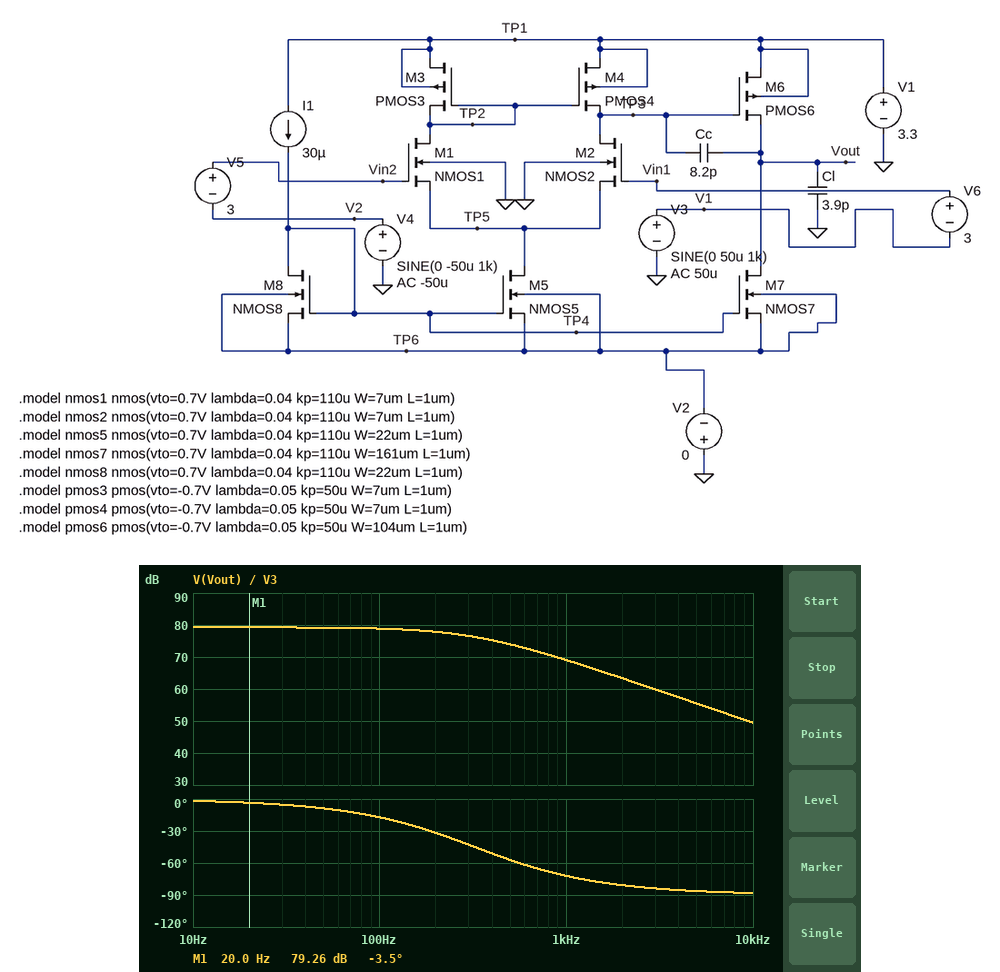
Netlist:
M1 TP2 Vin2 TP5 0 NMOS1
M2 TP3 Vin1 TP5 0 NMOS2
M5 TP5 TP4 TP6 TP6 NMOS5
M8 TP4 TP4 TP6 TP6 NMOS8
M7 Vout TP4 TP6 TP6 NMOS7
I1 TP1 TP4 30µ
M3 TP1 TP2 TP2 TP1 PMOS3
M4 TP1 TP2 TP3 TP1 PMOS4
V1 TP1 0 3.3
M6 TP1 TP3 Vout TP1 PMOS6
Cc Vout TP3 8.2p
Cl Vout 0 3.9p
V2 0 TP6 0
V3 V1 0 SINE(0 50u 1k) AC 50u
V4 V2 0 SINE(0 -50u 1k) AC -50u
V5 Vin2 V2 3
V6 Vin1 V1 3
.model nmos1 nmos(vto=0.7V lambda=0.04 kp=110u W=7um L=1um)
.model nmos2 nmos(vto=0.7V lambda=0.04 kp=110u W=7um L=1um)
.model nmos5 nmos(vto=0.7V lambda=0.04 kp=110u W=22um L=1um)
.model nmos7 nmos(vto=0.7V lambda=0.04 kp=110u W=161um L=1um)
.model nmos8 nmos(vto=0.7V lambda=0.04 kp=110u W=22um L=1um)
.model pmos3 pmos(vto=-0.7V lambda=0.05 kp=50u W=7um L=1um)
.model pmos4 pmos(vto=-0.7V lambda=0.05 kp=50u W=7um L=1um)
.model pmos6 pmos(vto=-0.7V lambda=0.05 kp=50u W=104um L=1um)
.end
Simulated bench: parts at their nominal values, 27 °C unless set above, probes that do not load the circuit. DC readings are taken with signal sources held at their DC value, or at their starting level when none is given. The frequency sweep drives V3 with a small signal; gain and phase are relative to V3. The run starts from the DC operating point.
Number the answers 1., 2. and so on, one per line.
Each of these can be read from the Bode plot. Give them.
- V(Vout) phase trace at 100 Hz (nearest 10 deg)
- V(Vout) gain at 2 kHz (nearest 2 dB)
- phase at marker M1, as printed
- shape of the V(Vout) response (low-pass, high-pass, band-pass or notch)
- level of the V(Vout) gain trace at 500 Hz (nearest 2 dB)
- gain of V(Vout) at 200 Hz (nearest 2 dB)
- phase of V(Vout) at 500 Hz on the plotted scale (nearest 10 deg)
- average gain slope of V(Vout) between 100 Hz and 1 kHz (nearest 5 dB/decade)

1. -20 deg
2. 64 dB
3. -3.5 deg
4. low-pass
5. 74 dB
6. 78 dB
7. -60 deg
8. -10 dB/decade
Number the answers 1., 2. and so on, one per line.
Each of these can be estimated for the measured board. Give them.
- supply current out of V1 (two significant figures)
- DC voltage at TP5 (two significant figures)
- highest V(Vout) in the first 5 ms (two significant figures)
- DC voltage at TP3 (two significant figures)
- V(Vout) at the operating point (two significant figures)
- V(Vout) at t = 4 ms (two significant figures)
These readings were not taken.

1. 290 µA
2. 2.1 V
3. 2.8 V
4. 2.3 V
5. 2.4 V
6. 2.1 V
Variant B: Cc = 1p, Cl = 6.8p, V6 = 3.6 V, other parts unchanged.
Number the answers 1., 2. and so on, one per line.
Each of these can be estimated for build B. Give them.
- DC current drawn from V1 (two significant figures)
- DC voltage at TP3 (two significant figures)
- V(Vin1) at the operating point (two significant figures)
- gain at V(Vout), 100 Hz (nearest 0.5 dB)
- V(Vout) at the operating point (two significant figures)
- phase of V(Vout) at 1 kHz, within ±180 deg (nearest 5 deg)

1. 300 µA
2. 2.1 V
3. 3.6 V
4. -40.0 dB
5. 3.2 V
6. 0 deg
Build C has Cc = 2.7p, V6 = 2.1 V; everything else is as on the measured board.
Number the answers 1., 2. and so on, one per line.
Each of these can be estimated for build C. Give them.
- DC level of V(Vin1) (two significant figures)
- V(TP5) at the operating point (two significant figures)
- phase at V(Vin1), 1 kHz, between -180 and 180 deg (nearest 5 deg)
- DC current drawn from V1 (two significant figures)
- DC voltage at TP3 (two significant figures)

1. 2.1 V
2. 2.0 V
3. 0 deg
4. 61 µA
5. 3.3 V
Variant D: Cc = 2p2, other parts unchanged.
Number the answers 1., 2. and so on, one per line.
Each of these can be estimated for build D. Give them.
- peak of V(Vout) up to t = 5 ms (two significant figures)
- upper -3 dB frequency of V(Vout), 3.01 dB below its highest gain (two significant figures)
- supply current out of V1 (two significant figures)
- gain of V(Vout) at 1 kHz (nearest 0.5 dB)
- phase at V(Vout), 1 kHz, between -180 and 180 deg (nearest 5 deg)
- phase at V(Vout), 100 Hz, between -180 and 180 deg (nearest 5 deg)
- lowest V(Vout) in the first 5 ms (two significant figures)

1. 3.0 V
2. 1.2 kHz
3. 290 µA
4. 77.0 dB
5. -40 deg
6. -5 deg
7. 1.7 V
